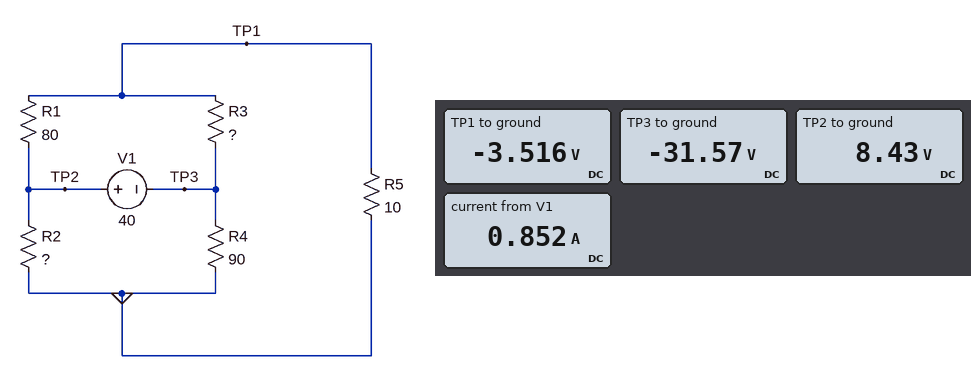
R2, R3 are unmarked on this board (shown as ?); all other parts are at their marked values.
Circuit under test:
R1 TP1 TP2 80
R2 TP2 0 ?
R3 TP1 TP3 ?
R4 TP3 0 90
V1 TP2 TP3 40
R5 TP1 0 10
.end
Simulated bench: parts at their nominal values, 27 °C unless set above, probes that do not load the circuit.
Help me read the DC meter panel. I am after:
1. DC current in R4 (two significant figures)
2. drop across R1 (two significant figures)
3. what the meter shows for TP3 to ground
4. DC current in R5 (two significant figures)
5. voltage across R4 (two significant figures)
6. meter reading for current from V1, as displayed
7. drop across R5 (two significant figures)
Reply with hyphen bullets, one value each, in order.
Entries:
- 350 mA
- 12 V
- -31.57 V
- 350 mA
- 32 V
- 0.852 A
- 3.5 V
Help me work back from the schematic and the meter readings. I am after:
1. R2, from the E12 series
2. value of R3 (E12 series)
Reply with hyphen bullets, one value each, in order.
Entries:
- 12 Ω
- 56 Ω
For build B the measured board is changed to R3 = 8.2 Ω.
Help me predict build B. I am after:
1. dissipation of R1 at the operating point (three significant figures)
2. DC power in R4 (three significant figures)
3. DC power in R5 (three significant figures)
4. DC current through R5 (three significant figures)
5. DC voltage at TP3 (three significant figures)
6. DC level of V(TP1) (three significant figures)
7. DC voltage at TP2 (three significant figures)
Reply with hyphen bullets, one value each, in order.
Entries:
- 9.73 W
- 6.07 W
- 12.7 W
- 1.13 A
- -23.4 V
- -11.3 V
- 16.6 V
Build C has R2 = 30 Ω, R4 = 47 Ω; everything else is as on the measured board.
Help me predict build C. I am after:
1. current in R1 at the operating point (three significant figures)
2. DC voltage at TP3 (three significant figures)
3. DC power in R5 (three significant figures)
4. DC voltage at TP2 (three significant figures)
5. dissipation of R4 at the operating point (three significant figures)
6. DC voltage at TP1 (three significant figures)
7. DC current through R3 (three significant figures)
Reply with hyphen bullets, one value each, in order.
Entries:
- 241 mA
- -22.0 V
- 168 mW
- 18.0 V
- 10.3 W
- -1.30 V
- 370 mA
